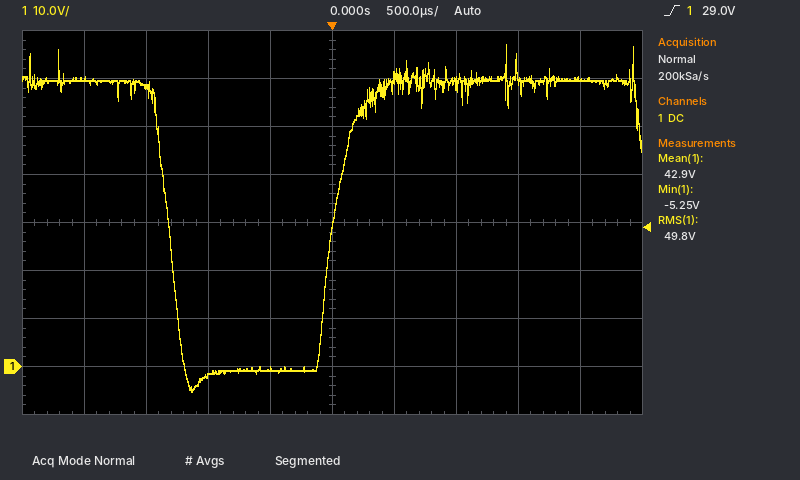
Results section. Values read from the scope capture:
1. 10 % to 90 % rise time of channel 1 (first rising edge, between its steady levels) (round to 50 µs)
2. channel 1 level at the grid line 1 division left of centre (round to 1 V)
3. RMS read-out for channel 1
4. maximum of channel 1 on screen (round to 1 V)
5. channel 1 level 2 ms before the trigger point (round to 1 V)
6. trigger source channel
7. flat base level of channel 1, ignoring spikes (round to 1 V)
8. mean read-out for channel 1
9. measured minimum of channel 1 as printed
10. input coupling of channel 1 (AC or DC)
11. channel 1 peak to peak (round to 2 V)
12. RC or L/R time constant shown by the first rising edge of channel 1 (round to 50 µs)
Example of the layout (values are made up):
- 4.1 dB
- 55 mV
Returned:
- 350 µs
- 0 V
- 49.8 V
- 67 V
- 60 V
- channel 1
- -1 V
- 42.9 V
- -5.25 V
- DC
- 72 V
- 150 µs
